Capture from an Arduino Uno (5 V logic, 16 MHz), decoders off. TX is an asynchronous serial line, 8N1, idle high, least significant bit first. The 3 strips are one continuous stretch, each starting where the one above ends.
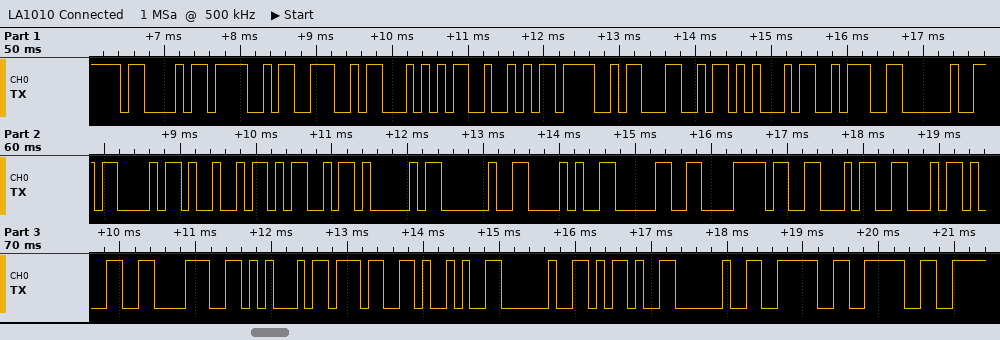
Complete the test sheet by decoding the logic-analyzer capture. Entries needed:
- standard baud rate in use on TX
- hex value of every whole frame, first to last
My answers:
9600 baud
43 4F 4E 54 52 4F 4C 45 3A 20 43 49 4D 41 20 28 30 78 46 46 31 38 45 37 29 20 2D 20 3E 3E
